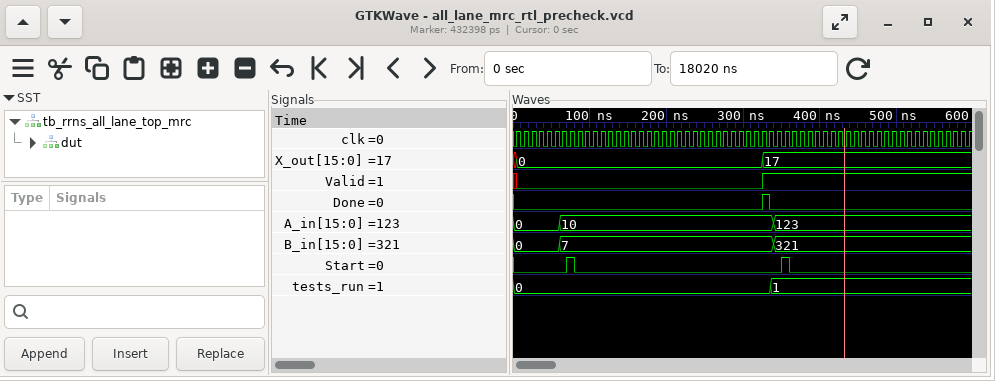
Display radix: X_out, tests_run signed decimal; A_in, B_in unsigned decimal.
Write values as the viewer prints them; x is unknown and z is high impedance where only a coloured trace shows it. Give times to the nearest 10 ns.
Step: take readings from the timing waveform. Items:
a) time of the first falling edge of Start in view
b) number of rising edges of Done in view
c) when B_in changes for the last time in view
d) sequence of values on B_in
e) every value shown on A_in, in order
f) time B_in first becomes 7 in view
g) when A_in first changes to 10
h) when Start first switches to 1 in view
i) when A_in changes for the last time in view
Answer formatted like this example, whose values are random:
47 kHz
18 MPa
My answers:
80 ns
1
340 ns
0, 7, 321
0, 10, 123
60 ns
60 ns
70 ns
340 ns
